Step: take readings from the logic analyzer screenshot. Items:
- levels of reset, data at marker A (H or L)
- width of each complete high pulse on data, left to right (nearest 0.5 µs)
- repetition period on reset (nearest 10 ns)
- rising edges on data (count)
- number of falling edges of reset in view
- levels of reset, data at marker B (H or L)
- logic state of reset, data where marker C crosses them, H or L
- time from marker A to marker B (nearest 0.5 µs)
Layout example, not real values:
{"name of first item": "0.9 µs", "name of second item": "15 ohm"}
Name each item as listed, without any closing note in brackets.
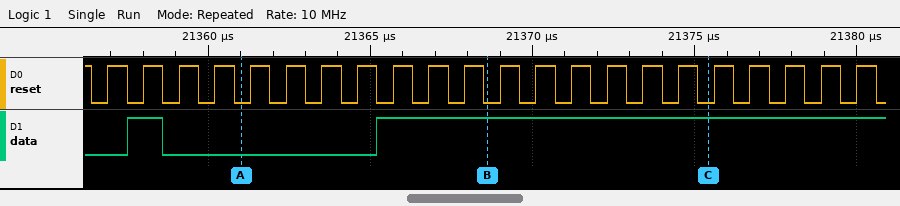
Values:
{"levels of reset, data at marker A": "reset=L, data=L", "width of each complete high pulse on data, left to right": "1 µs", "repetition period on reset": "1100 ns", "rising edges on data": "2", "number of falling edges of reset in view": "23", "levels of reset, data at marker B": "reset=L, data=H", "logic state of reset, data where marker C crosses them, H or L": "reset=L, data=H", "time from marker A to marker B": "7.5 µs"}
